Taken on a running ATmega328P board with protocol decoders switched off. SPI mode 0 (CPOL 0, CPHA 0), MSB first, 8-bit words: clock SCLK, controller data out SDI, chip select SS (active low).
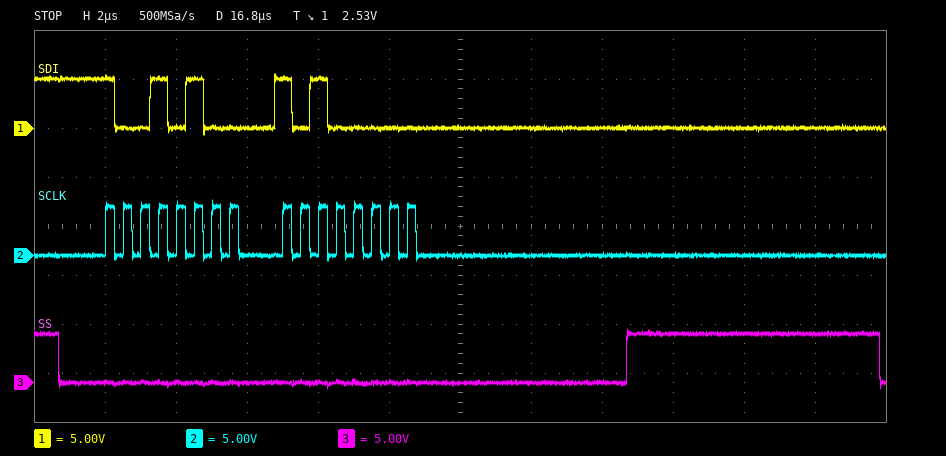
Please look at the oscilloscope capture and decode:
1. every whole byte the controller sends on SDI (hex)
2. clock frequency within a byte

94 A0
2 MHz
